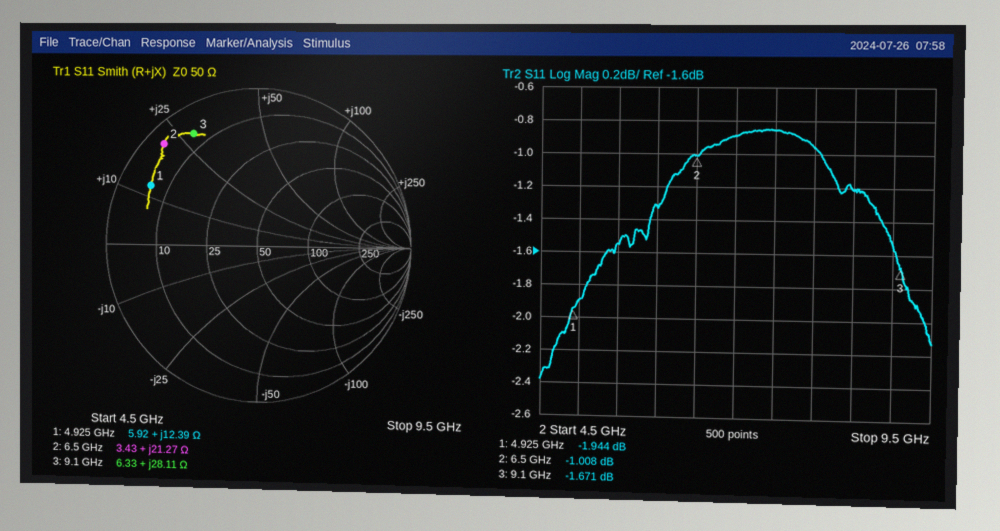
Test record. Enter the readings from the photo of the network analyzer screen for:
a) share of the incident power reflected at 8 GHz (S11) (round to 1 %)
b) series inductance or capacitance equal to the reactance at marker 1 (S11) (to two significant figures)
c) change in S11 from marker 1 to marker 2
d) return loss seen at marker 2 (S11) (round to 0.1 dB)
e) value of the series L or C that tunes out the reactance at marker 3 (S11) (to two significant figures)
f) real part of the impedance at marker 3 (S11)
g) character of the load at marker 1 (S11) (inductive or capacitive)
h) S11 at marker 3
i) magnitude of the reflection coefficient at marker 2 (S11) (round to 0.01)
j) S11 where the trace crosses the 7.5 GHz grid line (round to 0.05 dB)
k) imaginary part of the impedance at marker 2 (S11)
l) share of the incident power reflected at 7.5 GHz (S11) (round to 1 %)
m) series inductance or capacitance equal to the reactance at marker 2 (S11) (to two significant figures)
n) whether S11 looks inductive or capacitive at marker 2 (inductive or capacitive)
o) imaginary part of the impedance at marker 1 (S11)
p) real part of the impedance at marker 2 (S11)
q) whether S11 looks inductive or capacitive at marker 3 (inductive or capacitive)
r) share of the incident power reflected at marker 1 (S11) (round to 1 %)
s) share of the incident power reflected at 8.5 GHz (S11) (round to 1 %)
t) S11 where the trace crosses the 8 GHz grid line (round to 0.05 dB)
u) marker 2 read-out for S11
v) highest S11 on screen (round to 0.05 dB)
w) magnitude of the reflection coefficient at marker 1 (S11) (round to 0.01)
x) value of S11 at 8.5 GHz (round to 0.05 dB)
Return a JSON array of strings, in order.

["80 %", "400 pH", "0.936 dB", "1.0 dB", "620 fF", "6.33 Ω", "inductive", "-1.671 dB", "0.89", "-0.85 dB", "+21.27 Ω", "82 %", "520 pH", "inductive", "+12.39 Ω", "3.43 Ω", "inductive", "64 %", "76 %", "-0.95 dB", "-1.008 dB", "-0.85 dB", "0.80", "-1.20 dB"]
